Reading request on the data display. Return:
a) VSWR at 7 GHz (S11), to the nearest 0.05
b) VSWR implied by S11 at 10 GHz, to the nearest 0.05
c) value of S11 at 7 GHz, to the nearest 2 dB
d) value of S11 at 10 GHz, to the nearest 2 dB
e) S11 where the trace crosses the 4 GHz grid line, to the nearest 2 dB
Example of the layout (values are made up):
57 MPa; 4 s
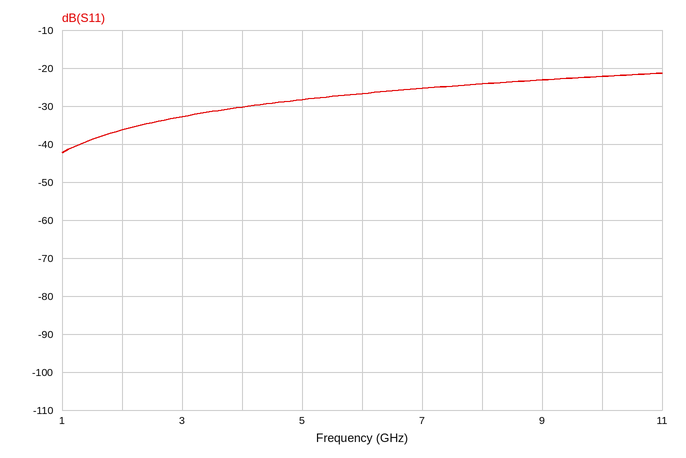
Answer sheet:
1.10; 1.15; -26 dB; -22 dB; -30 dB
